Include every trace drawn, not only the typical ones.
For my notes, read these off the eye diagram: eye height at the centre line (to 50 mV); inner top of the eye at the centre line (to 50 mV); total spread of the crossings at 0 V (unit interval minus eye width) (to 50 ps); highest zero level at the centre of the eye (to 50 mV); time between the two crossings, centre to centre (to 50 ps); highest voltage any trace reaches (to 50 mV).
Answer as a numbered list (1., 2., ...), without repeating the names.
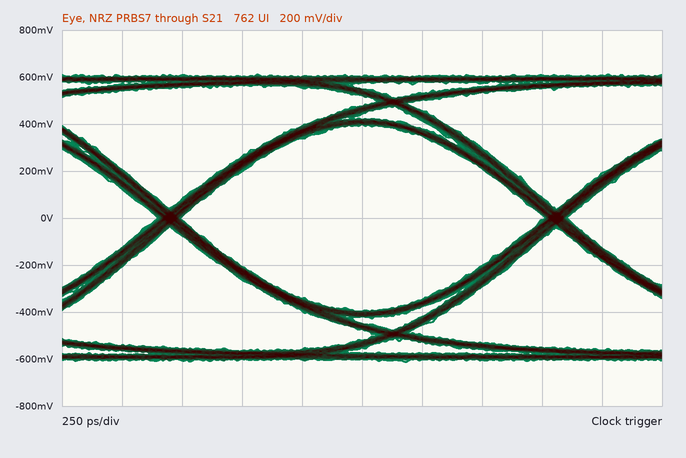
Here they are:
1. 800 mV
2. 400 mV
3. 100 ps
4. -400 mV
5. 1.60 ns
6. 600 mV
